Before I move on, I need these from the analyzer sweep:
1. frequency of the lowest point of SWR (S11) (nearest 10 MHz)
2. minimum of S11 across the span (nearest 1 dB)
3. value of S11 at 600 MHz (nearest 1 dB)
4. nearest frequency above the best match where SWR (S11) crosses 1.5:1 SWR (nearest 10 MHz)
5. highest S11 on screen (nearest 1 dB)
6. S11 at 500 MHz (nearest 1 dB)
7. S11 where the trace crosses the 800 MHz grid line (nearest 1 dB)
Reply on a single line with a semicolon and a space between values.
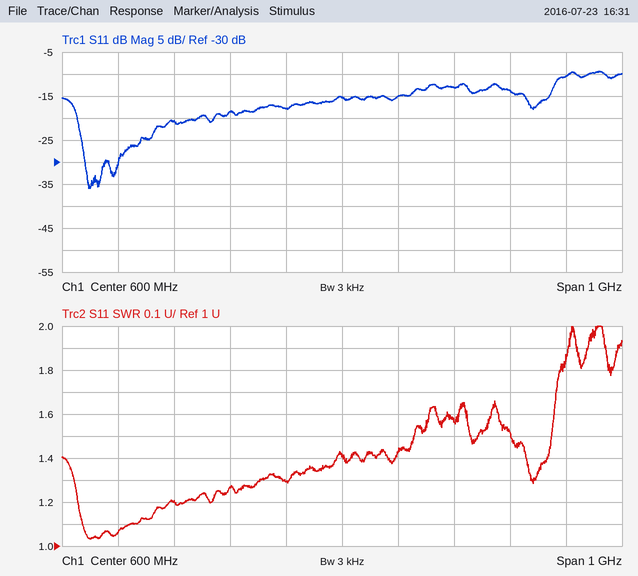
150 MHz; -36 dB; -15 dB; 730 MHz; -9 dB; -18 dB; -13 dB
